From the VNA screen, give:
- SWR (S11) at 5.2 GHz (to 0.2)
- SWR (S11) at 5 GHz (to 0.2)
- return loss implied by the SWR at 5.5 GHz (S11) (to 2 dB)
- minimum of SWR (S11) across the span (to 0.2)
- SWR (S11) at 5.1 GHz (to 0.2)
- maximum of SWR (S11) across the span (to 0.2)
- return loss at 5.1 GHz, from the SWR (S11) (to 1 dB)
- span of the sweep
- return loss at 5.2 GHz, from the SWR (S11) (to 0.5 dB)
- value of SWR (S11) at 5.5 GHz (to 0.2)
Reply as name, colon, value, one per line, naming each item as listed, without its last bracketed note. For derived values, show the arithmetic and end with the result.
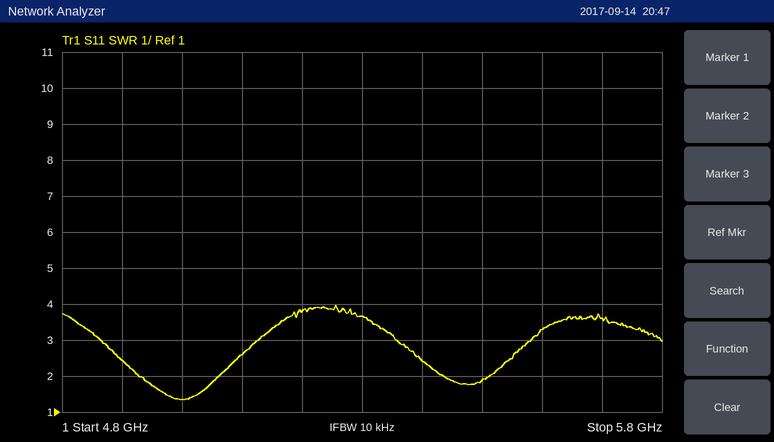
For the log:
SWR (S11) at 5.2 GHz: 3.8
SWR (S11) at 5 GHz: 1.4
return loss implied by the SWR at 5.5 GHz (S11): −20 log10((1.8 − 1)/(1.8 + 1)) ≈ 10.9 dB, so 10 dB to the nearest 2 dB
minimum of SWR (S11) across the span: 1.4
SWR (S11) at 5.1 GHz: 2.6
maximum of SWR (S11) across the span: 4.0
return loss at 5.1 GHz, from the SWR (S11): −20 log10((2.6 − 1)/(2.6 + 1)) ≈ 7 dB
span of the sweep: 1 GHz
return loss at 5.2 GHz, from the SWR (S11): −20 log10((3.8 − 1)/(3.8 + 1)) ≈ 4.68 dB, so 4.5 dB to the nearest 0.5 dB
value of SWR (S11) at 5.5 GHz: 1.8
